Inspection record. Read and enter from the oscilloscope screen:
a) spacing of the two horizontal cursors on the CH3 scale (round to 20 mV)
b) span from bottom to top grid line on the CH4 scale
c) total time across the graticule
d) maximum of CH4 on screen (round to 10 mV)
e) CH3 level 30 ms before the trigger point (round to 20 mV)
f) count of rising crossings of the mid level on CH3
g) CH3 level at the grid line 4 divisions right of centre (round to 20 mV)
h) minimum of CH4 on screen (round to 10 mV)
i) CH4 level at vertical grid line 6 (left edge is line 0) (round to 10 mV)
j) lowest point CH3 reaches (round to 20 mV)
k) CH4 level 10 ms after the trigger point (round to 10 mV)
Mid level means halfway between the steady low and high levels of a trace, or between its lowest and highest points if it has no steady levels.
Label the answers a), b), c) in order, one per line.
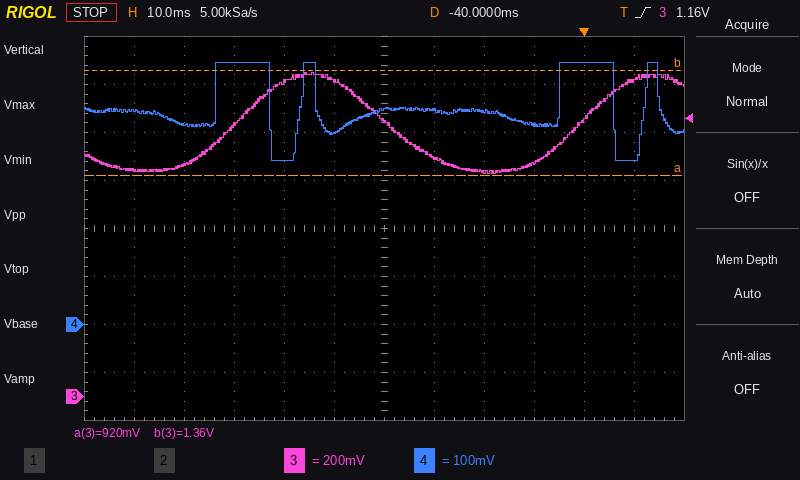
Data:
a) 440 mV
b) 800 mV
c) 120 ms
d) 550 mV
e) 1.00 V
f) 2
g) 1.16 V
h) 340 mV
i) 450 mV
j) 920 mV
k) 340 mV
